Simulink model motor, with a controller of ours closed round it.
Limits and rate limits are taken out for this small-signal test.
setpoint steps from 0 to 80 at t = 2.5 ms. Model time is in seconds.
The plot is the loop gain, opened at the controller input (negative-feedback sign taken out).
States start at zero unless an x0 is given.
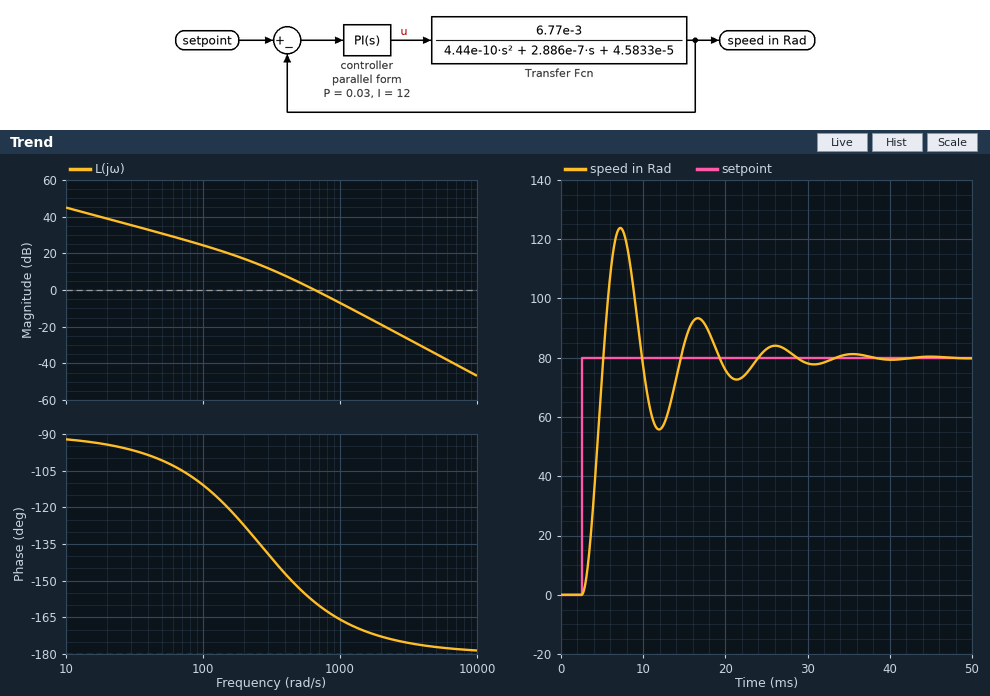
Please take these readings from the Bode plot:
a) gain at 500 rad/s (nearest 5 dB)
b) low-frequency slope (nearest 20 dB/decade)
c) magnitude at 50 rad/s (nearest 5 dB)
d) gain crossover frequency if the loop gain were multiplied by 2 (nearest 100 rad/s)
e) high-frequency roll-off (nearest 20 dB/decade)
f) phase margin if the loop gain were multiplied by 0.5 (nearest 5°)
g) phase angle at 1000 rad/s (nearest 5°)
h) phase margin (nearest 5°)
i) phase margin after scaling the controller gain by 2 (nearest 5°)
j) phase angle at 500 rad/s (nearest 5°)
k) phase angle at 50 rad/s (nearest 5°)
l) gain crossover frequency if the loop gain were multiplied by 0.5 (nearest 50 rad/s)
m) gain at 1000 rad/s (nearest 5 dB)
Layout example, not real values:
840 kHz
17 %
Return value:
5 dB
-20 dB/decade
30 dB
900 rad/s
-40 dB/decade
30°
-165°
20°
15°
-155°
-100°
450 rad/s
-5 dB
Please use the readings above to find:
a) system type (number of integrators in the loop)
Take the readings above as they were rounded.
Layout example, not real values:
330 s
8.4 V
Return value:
1
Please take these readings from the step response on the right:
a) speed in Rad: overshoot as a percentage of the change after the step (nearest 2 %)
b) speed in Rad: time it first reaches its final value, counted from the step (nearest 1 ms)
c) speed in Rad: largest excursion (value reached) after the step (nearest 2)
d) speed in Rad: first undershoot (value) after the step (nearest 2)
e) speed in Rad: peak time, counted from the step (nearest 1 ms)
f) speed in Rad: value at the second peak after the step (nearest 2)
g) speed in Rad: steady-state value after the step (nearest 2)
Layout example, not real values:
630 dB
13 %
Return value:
54 %
3 ms
124
56
5 ms
94
80
